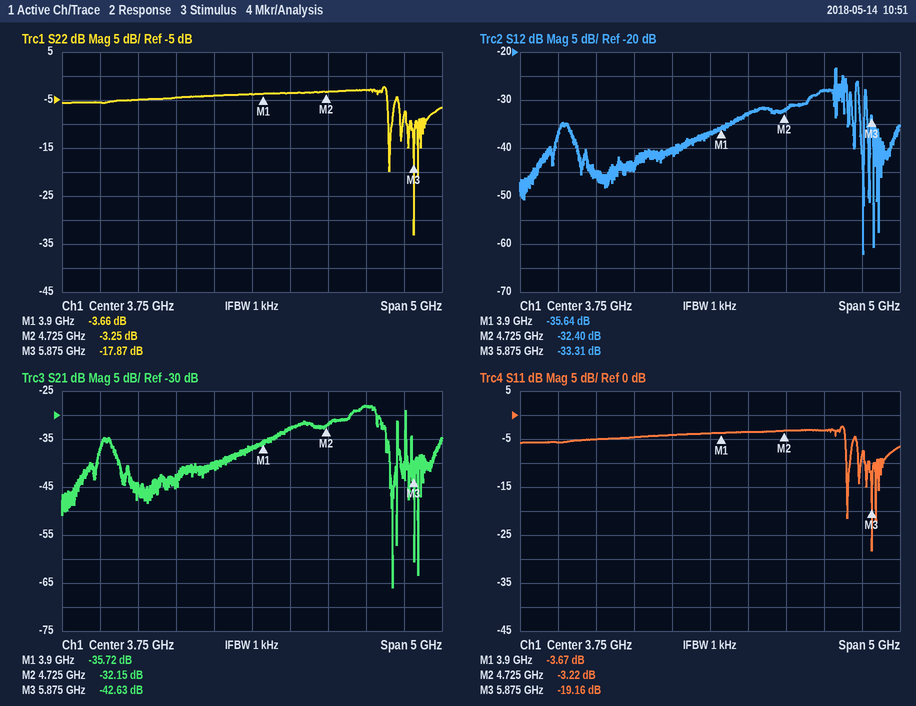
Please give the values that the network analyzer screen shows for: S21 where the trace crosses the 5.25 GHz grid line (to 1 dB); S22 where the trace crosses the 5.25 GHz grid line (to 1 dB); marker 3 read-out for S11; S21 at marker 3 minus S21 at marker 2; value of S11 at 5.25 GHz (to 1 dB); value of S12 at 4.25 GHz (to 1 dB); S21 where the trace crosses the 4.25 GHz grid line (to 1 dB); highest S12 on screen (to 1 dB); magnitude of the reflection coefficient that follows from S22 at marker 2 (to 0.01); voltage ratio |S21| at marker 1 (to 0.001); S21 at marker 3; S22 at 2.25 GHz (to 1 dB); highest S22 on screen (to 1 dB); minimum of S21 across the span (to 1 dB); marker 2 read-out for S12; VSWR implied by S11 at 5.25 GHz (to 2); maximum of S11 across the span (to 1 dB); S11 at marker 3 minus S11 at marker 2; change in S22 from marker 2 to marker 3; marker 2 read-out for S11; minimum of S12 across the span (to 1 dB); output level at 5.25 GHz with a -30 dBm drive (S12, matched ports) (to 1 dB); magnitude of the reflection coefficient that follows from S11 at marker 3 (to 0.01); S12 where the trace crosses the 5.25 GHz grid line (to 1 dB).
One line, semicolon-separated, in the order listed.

-28 dB; -3 dB; -19.16 dB; -10.48 dB; -3 dB; -33 dB; -33 dB; -23 dB; 0.69; 0.016; -42.63 dB; -5 dB; -2 dB; -66 dB; -32.40 dB; 6; -2 dB; -15.94 dB; -14.62 dB; -3.22 dB; -62 dB; -58 dBm; 0.11; -28 dB
